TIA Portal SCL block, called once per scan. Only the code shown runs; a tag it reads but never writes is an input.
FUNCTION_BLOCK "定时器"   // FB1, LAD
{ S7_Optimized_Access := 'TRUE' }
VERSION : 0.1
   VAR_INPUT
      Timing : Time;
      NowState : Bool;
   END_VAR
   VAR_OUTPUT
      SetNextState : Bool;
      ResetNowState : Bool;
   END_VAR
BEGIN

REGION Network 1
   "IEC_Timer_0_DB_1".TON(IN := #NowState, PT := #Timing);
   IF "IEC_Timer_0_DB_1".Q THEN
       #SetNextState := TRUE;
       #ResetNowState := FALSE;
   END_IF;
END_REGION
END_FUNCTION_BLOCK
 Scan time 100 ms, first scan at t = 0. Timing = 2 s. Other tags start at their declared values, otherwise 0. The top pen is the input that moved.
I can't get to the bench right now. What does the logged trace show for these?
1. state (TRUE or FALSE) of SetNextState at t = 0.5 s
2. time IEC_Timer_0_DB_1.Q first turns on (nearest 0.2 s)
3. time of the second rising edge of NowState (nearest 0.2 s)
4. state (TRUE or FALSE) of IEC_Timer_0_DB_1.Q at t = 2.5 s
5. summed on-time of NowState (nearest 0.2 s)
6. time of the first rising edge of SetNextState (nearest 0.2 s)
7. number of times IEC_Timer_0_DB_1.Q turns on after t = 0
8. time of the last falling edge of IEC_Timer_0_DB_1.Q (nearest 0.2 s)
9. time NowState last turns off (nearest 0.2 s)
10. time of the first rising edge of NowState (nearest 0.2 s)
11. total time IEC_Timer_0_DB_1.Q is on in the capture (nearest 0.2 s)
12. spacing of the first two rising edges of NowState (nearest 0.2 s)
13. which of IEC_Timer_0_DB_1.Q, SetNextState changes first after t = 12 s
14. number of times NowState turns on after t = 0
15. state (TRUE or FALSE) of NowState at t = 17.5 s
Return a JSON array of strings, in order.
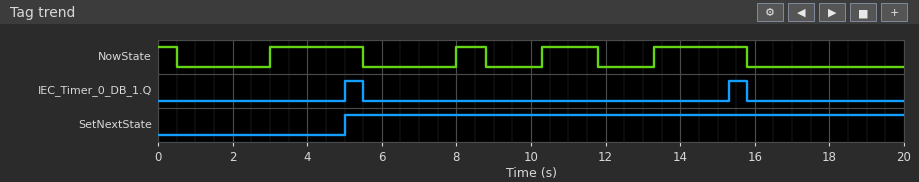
["FALSE", "5.0 s", "8.0 s", "FALSE", "7.8 s", "5.0 s", "2", "15.8 s", "15.8 s", "3.0 s", "1.0 s", "5.0 s", "IEC_Timer_0_DB_1.Q", "4", "FALSE"]
